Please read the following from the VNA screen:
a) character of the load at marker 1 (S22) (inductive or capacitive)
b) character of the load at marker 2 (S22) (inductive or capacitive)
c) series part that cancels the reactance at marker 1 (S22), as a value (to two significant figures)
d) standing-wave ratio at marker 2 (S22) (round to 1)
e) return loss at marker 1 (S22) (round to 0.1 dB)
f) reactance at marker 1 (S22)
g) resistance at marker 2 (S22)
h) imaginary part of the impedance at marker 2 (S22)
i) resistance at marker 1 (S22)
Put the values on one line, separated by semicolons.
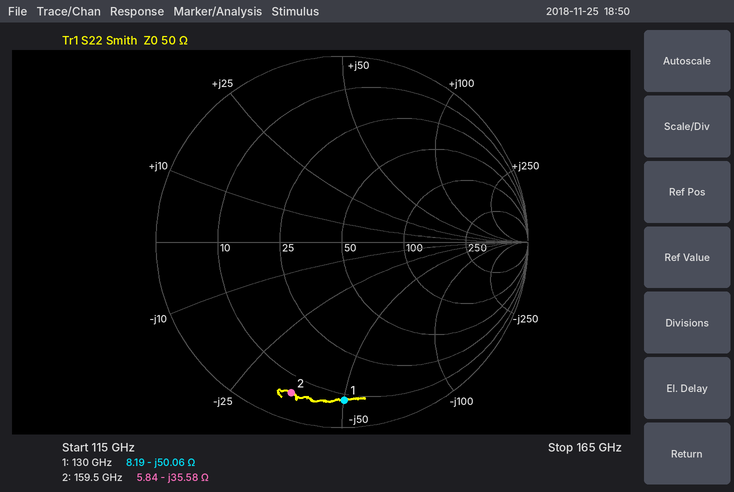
capacitive; capacitive; 61 pH; 13; 1.4 dB; -50.06 Ω; 5.84 Ω; -35.58 Ω; 8.19 Ω
